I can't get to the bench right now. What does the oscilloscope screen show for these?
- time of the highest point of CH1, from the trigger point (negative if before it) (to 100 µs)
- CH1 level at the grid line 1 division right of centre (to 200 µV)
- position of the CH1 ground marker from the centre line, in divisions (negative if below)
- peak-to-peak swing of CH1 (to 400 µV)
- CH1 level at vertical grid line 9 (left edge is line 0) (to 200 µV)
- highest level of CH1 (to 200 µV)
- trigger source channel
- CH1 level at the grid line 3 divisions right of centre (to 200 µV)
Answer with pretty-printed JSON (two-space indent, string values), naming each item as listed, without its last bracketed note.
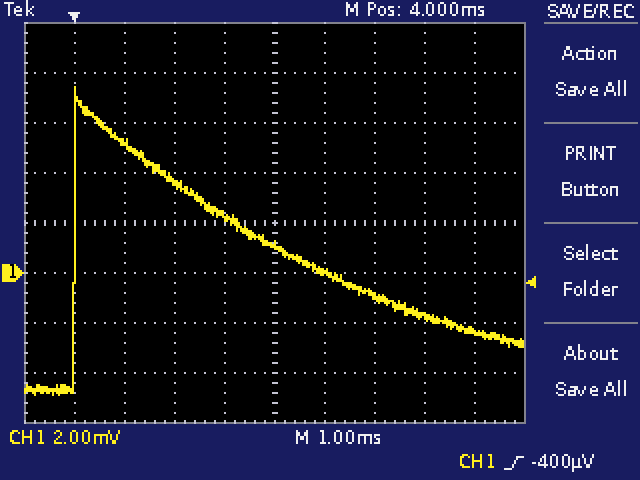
{
  "time of the highest point of CH1, from the trigger point (negative if before it)": "0.0 ms",
  "CH1 level at the grid line 1 division right of centre": "0.0 mV",
  "position of the CH1 ground marker from the centre line, in divisions": "-1.0 div",
  "peak-to-peak swing of CH1": "12.4 mV",
  "CH1 level at vertical grid line 9 (left edge is line 0)": "-2.4 mV",
  "highest level of CH1": "7.4 mV",
  "trigger source channel": "CH1",
  "CH1 level at the grid line 3 divisions right of centre": "-1.8 mV"
}
